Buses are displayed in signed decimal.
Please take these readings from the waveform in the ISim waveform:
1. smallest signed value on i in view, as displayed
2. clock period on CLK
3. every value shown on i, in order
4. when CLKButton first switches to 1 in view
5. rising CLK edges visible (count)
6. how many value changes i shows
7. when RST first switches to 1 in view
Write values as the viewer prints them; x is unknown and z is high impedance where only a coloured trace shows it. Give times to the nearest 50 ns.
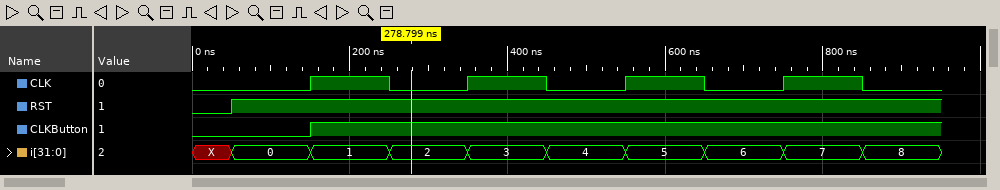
0
200 ns
X, 0, 1, 2, 3, 4, 5, 6, 7, 8
150 ns
4
9
50 ns
